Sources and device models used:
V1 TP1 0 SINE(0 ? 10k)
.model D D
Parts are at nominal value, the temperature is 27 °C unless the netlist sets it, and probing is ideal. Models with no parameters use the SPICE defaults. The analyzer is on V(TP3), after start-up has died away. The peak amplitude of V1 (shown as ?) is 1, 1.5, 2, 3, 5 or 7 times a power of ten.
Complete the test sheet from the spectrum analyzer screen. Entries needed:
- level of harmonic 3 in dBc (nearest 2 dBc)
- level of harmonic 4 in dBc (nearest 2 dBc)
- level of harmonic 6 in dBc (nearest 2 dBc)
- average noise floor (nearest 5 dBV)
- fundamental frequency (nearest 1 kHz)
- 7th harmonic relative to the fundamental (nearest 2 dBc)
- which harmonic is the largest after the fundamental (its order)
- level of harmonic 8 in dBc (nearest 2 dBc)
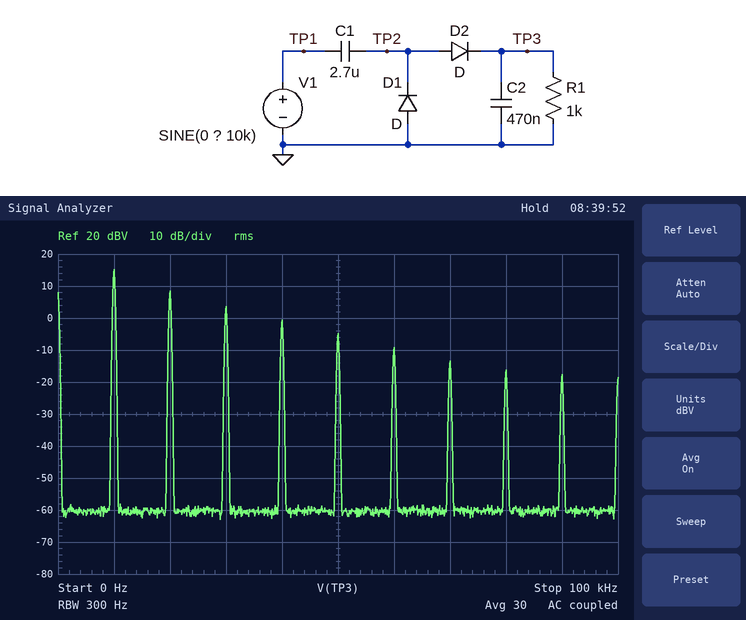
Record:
-12 dBc
-16 dBc
-24 dBc
-60 dBV
10 kHz
-28 dBc
2
-32 dBc
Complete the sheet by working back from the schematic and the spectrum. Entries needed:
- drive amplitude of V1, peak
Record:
70 V
